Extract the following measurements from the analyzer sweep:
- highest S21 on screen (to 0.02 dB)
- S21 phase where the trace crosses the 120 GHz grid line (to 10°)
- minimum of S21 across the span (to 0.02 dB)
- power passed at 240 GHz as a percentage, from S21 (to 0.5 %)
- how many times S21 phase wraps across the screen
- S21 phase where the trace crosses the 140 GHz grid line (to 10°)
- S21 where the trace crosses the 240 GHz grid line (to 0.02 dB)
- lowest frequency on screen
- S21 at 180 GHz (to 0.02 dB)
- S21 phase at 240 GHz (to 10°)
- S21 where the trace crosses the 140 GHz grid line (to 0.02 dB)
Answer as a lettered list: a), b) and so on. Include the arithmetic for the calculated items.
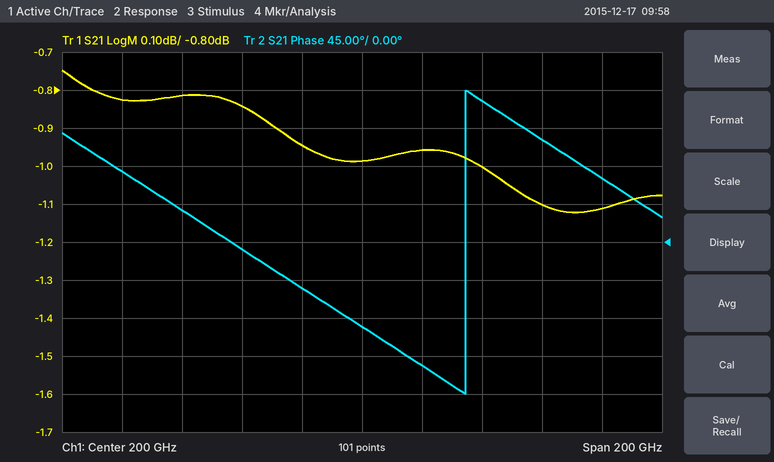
a) -0.74 dB
b) 80°
c) -1.12 dB
d) 10^(-1/10) ≈ 79.4 %, so 79.5 % to the nearest 0.5 %
e) 1
f) 40°
g) -1.00 dB
h) 100 GHz
i) -0.94 dB
j) 170°
k) -0.82 dB
